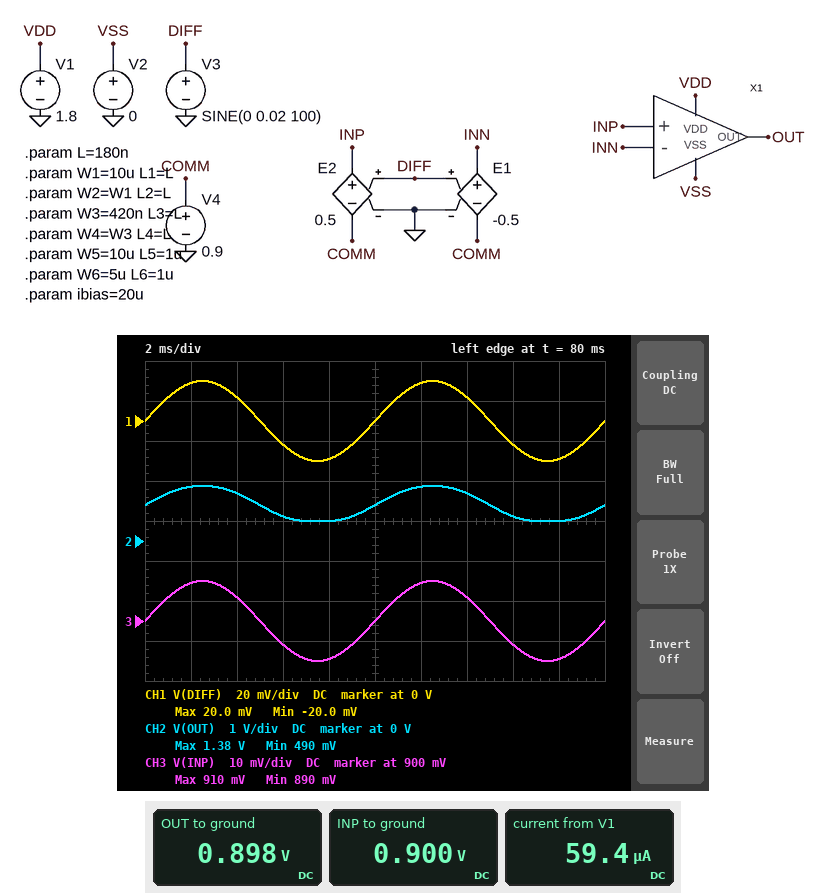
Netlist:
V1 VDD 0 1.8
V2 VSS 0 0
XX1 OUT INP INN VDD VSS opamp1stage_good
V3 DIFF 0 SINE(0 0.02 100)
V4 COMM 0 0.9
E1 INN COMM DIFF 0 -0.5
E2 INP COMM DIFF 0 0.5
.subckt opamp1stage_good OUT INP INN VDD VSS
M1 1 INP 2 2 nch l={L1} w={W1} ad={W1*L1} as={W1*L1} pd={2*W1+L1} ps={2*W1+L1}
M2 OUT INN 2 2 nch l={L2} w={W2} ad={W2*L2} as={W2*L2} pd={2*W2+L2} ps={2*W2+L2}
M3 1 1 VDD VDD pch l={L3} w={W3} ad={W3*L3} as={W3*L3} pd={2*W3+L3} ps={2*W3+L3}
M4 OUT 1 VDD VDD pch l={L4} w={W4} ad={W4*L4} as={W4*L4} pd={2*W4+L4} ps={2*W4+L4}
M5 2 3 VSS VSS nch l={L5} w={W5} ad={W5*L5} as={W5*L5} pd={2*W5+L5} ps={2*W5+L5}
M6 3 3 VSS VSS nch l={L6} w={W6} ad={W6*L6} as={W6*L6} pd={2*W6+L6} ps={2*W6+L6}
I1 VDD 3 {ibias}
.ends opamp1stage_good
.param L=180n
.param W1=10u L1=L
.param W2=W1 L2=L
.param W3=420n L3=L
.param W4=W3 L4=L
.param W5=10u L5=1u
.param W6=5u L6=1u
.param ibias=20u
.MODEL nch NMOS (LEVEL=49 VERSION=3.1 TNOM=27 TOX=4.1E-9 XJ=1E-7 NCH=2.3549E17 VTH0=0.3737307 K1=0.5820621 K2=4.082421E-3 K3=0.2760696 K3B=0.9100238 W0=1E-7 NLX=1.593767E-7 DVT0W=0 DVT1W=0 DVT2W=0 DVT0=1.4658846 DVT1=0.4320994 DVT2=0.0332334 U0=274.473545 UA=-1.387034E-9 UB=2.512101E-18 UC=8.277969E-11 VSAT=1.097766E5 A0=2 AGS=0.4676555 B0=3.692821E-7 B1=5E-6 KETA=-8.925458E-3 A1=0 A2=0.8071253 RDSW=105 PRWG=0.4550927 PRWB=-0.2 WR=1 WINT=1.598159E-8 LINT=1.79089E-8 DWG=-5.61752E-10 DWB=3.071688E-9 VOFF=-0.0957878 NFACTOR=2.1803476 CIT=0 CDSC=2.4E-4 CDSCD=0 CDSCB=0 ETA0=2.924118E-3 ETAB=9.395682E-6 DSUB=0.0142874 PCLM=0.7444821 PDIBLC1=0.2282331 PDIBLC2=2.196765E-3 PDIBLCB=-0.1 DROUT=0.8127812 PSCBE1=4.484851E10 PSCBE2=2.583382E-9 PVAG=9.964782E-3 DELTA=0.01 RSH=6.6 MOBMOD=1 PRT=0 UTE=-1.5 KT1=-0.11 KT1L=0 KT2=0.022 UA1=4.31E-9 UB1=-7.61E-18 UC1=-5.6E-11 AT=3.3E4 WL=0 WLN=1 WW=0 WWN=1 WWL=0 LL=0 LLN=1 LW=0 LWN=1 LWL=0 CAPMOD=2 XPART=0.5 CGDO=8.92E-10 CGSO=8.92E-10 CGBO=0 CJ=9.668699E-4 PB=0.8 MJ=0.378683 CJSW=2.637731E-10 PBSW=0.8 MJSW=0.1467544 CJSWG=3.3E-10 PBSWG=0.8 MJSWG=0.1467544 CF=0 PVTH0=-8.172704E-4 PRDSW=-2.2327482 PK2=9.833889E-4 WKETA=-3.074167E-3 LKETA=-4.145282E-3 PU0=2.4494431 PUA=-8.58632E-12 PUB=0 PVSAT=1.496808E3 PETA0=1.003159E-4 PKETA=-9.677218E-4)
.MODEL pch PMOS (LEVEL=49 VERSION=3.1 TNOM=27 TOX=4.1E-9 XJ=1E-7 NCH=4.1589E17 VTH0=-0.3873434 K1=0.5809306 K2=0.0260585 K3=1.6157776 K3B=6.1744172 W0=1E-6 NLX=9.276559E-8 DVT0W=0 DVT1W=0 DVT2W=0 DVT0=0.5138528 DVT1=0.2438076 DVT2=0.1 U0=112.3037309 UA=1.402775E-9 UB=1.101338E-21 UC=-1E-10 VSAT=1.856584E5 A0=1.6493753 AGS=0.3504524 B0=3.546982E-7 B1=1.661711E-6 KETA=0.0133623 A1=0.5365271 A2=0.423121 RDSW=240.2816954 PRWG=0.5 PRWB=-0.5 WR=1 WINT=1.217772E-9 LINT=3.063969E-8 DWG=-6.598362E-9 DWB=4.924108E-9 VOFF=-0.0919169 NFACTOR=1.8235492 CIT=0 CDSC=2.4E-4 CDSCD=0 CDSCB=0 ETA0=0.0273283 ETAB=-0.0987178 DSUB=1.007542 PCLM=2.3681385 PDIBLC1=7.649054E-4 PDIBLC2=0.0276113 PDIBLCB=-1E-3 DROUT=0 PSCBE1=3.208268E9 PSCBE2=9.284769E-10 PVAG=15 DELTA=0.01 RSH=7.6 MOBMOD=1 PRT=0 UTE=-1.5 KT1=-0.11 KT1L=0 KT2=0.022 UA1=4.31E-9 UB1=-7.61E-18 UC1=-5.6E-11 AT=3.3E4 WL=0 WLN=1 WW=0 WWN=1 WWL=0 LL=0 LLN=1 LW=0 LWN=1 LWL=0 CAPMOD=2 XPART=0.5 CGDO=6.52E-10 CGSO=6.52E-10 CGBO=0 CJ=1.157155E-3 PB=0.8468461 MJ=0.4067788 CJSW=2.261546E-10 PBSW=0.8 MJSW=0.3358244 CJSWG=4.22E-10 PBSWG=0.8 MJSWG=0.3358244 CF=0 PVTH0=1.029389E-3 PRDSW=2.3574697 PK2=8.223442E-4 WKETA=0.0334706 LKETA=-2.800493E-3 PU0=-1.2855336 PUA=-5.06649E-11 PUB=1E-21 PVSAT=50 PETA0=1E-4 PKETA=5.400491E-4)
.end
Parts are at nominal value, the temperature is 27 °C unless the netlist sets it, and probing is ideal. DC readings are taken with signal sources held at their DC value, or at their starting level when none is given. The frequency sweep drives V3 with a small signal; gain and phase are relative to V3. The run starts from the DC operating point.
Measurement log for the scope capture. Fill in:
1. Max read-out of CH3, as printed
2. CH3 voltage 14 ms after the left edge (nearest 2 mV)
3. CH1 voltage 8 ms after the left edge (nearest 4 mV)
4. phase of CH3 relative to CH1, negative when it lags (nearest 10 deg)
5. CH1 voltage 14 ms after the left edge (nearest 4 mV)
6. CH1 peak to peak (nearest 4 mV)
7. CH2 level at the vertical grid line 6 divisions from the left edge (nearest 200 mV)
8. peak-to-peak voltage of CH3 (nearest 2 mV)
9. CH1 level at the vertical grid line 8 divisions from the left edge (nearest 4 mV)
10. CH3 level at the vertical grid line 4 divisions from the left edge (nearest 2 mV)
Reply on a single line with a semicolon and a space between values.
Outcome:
910 mV; 906 mV; -20 mV; 0 deg; 12 mV; 40 mV; 1.4 V; 20 mV; -12 mV; 890 mV
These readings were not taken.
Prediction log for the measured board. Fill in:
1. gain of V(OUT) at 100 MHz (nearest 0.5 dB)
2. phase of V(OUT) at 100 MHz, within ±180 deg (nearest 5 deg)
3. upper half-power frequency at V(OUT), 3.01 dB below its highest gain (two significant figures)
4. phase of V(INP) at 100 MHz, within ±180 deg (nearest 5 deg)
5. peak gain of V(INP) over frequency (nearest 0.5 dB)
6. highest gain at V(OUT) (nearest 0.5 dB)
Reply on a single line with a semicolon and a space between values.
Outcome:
26.5 dB; -35 deg; 150 MHz; 0 deg; -6.0 dB; 28.0 dB
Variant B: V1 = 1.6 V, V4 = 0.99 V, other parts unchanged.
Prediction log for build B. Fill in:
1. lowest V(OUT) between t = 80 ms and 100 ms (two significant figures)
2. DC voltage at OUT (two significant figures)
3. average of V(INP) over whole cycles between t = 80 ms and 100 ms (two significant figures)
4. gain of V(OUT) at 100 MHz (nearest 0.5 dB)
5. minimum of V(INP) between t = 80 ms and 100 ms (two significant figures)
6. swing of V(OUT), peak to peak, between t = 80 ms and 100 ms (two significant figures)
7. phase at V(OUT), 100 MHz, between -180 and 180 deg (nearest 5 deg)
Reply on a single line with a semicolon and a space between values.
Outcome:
530 mV; 700 mV; 990 mV; 25.0 dB; 980 mV; 610 mV; -30 deg
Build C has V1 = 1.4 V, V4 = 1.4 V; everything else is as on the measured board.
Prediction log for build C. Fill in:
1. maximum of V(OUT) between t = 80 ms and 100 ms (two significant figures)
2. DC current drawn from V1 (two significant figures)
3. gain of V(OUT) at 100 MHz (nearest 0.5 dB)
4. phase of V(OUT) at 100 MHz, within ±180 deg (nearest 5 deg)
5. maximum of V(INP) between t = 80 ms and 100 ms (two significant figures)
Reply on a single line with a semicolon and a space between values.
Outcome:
500 mV; 60 µA; -45.0 dB; -25 deg; 1.4 V
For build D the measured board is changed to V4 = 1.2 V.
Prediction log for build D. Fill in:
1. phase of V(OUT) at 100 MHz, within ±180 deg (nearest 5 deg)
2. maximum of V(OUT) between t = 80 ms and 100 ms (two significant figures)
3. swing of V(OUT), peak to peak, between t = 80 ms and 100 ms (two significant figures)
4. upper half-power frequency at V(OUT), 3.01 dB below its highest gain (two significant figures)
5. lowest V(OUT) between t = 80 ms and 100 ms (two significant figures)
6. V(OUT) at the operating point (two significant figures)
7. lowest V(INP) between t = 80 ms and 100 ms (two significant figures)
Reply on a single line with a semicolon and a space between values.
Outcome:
-30 deg; 1.3 V; 590 mV; 190 MHz; 740 mV; 890 mV; 1.2 V
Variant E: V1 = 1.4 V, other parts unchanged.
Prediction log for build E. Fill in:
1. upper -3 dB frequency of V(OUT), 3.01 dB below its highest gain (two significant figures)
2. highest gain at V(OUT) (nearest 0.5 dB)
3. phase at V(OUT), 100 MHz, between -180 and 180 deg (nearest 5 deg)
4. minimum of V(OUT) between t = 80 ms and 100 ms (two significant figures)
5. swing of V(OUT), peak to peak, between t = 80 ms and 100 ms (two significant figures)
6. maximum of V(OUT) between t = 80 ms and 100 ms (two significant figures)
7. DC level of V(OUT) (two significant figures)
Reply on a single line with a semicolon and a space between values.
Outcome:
340 MHz; 20.0 dB; -20 deg; 430 mV; 440 mV; 870 mV; 500 mV
